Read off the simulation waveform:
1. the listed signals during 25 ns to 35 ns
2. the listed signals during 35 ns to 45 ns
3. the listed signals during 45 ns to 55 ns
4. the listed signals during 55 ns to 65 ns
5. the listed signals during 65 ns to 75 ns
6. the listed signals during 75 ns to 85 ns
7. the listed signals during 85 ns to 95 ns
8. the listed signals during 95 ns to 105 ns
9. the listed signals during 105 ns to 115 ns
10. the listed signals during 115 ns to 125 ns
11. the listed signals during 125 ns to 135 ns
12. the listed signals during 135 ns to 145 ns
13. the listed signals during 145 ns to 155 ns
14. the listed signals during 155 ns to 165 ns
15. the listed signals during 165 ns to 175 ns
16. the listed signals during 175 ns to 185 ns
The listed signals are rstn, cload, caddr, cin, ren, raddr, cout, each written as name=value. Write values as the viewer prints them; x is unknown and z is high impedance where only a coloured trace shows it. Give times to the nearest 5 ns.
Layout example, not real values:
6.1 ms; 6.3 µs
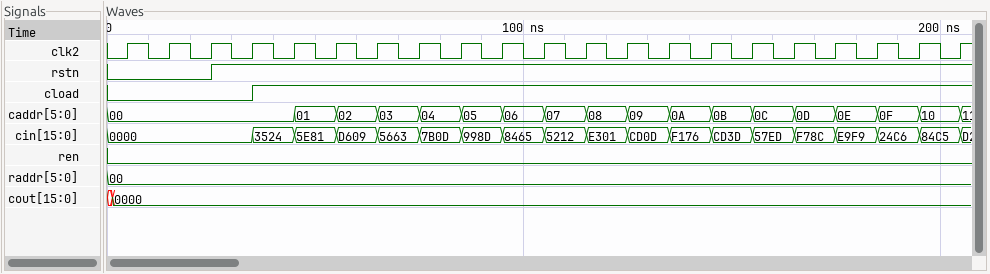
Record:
rstn=1, cload=0, caddr=00, cin=0000, ren=0, raddr=00, cout=0000; rstn=1, cload=1, caddr=00, cin=3524, ren=0, raddr=00, cout=0000; rstn=1, cload=1, caddr=01, cin=5E81, ren=0, raddr=00, cout=0000; rstn=1, cload=1, caddr=02, cin=D609, ren=0, raddr=00, cout=0000; rstn=1, cload=1, caddr=03, cin=5663, ren=0, raddr=00, cout=0000; rstn=1, cload=1, caddr=04, cin=7B0D, ren=0, raddr=00, cout=0000; rstn=1, cload=1, caddr=05, cin=998D, ren=0, raddr=00, cout=0000; rstn=1, cload=1, caddr=06, cin=8465, ren=0, raddr=00, cout=0000; rstn=1, cload=1, caddr=07, cin=5212, ren=0, raddr=00, cout=0000; rstn=1, cload=1, caddr=08, cin=E301, ren=0, raddr=00, cout=0000; rstn=1, cload=1, caddr=09, cin=CD0D, ren=0, raddr=00, cout=0000; rstn=1, cload=1, caddr=0A, cin=F176, ren=0, raddr=00, cout=0000; rstn=1, cload=1, caddr=0B, cin=CD3D, ren=0, raddr=00, cout=0000; rstn=1, cload=1, caddr=0C, cin=57ED, ren=0, raddr=00, cout=0000; rstn=1, cload=1, caddr=0D, cin=F78C, ren=0, raddr=00, cout=0000; rstn=1, cload=1, caddr=0E, cin=E9F9, ren=0, raddr=00, cout=0000
